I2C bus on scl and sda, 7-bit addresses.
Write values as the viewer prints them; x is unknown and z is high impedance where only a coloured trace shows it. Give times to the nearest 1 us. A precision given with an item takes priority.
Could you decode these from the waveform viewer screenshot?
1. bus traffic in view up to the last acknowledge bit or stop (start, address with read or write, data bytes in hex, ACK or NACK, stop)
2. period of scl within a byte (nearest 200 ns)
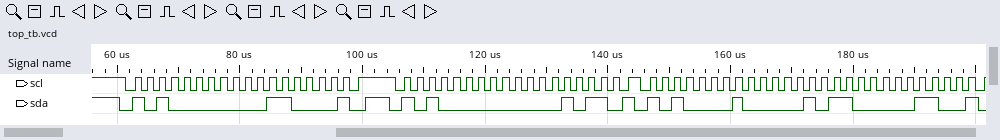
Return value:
start, address 50 write ACK, 30 NACK, stop, start, address 50 write ACK, 0B ACK, repeated start, address 50 read ACK, 0B ACK, 0C NACK
2000 ns
